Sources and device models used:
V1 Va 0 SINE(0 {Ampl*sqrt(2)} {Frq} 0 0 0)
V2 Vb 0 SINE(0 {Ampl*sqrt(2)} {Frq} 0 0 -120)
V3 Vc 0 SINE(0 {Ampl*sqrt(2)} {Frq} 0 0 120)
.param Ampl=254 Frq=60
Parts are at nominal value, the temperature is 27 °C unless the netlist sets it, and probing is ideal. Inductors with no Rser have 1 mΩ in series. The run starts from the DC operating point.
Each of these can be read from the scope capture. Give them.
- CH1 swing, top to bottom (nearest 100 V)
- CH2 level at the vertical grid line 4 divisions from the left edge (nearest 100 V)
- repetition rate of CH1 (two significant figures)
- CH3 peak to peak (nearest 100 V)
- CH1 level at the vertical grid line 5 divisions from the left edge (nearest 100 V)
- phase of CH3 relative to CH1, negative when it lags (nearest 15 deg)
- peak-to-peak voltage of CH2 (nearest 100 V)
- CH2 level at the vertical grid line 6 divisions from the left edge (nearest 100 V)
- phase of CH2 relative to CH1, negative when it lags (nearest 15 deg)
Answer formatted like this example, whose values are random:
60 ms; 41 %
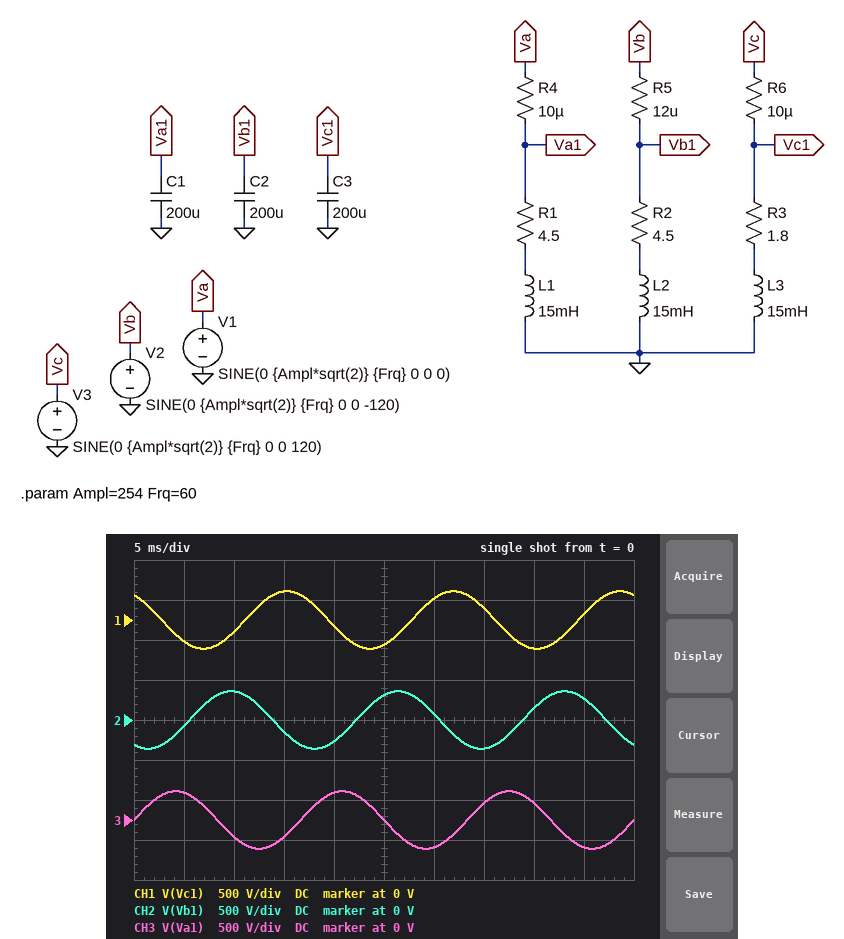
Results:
700 V; -300 V; 60 Hz; 700 V; -300 V; -120 deg; 700 V; 100 V; 120 deg
